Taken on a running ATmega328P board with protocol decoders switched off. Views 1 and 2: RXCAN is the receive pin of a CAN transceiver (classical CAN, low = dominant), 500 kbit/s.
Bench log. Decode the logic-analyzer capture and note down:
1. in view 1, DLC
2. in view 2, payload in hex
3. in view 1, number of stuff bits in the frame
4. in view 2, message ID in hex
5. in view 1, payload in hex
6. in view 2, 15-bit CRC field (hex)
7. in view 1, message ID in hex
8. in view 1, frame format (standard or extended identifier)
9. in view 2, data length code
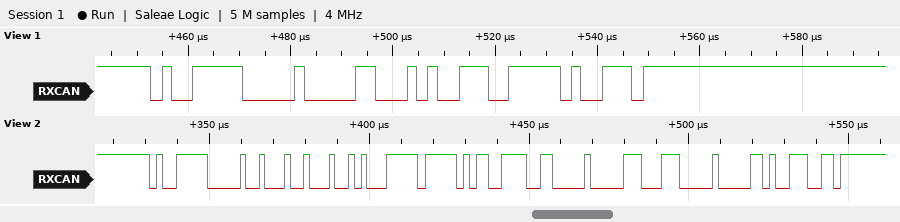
1
91 28 FF EC F3 00 31 C0
4
0x4F8
14
0x0539
0x4F8
standard
8
